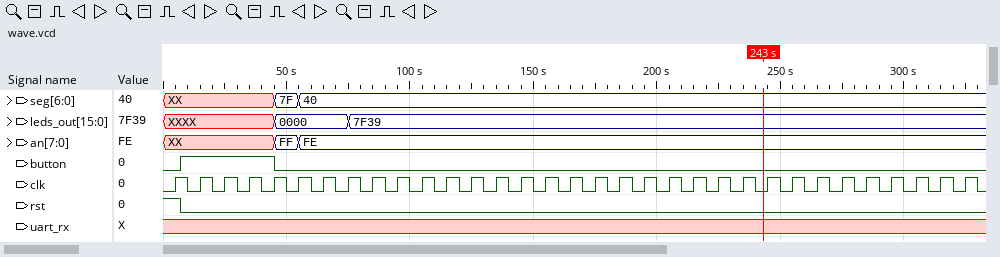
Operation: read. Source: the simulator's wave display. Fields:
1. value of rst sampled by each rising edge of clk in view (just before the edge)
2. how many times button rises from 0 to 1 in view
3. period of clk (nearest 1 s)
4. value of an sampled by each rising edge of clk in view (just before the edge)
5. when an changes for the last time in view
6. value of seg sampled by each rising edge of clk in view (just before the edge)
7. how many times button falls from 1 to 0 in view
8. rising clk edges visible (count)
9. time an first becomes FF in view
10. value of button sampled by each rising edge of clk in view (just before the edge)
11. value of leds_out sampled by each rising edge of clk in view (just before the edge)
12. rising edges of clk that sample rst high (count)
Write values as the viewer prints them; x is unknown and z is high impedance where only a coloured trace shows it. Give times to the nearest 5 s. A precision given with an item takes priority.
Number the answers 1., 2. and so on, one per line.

1. 1 0 0 0 0 0 0 0 0 0 0 0 0 0 0 0 0 0 0 0 0 0 0 0 0 0 0 0 0 0 0 0 0
2. 1
3. 10 s
4. XX, XX, XX, XX, XX, FF, FE, FE, FE, FE, FE, FE, FE, FE, FE, FE, FE, FE, FE, FE, FE, FE, FE, FE, FE, FE, FE, FE, FE, FE, FE, FE, FE
5. 55 s
6. XX, XX, XX, XX, XX, 7F, 40, 40, 40, 40, 40, 40, 40, 40, 40, 40, 40, 40, 40, 40, 40, 40, 40, 40, 40, 40, 40, 40, 40, 40, 40, 40, 40
7. 1
8. 33
9. 45 s
10. 0 1 1 1 1 0 0 0 0 0 0 0 0 0 0 0 0 0 0 0 0 0 0 0 0 0 0 0 0 0 0 0 0
11. XXXX, XXXX, XXXX, XXXX, XXXX, 0000, 0000, 0000, 7F39, 7F39, 7F39, 7F39, 7F39, 7F39, 7F39, 7F39, 7F39, 7F39, 7F39, 7F39, 7F39, 7F39, 7F39, 7F39, 7F39, 7F39, 7F39, 7F39, 7F39, 7F39, 7F39, 7F39, 7F39
12. 1
